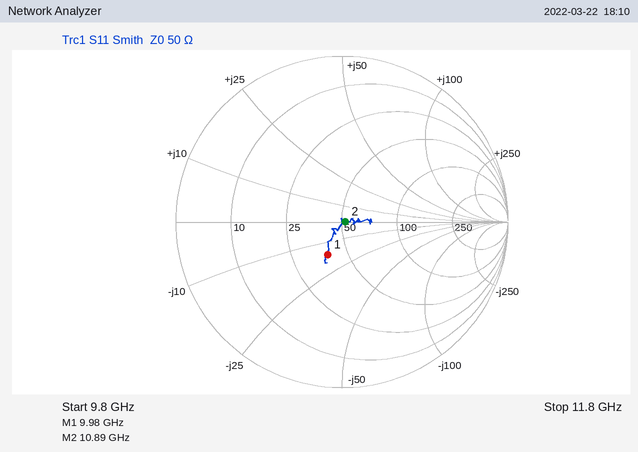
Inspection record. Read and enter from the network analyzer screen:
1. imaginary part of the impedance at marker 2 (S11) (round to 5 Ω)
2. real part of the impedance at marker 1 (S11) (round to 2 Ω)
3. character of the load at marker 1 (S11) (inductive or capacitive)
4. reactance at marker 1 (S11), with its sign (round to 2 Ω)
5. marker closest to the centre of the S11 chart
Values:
0 Ω
40 Ω
capacitive
-16 Ω
marker 2
